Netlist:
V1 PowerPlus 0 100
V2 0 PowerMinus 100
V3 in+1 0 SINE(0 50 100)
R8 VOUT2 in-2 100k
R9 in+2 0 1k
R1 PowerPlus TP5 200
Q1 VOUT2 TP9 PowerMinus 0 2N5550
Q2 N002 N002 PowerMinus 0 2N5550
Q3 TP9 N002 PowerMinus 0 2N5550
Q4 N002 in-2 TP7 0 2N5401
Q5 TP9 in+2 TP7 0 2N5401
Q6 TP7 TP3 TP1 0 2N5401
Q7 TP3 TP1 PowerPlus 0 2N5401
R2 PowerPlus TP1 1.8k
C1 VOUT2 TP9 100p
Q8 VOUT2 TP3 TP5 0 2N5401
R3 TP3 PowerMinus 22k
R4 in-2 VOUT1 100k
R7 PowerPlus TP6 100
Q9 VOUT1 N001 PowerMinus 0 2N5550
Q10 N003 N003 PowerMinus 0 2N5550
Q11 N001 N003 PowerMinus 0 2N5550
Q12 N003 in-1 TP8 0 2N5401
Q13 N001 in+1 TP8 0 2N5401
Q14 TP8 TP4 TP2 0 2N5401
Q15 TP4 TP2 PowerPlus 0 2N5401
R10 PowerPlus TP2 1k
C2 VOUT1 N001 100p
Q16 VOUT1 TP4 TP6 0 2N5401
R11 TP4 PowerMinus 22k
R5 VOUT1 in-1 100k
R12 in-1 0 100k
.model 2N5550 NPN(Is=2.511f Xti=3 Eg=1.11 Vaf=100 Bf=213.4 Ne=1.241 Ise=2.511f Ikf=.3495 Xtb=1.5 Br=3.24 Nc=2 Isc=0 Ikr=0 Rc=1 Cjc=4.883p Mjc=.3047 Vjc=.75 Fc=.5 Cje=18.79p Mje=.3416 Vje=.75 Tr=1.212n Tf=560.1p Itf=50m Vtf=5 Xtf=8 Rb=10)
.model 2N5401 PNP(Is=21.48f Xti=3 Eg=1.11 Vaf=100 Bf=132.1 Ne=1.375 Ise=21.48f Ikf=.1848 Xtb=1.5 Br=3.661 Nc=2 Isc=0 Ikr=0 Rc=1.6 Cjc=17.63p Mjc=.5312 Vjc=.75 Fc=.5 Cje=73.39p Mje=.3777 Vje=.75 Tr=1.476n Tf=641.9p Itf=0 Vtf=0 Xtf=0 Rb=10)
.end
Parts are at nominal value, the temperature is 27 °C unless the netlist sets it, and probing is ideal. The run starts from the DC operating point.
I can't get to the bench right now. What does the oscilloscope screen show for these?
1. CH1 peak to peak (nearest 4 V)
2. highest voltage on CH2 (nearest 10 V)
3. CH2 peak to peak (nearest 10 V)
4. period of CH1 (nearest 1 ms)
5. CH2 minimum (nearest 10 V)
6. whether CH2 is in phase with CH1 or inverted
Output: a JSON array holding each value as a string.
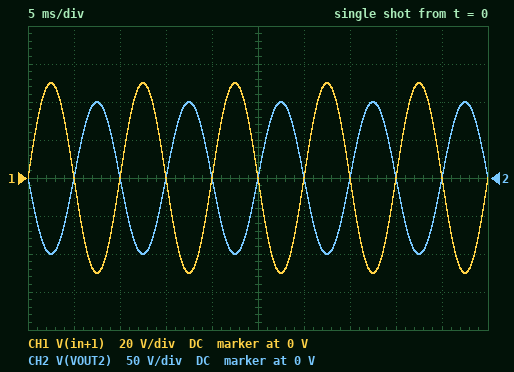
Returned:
["100 V", "100 V", "200 V", "10 ms", "-100 V", "inverted"]
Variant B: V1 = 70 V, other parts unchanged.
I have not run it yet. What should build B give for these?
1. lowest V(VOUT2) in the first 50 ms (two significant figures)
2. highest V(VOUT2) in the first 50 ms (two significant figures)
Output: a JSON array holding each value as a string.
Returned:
["-70 V", "69 V"]
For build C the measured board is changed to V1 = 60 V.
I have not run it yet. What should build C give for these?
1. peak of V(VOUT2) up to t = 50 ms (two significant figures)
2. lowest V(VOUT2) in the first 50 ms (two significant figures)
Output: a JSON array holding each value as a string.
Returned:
["59 V", "-60 V"]
